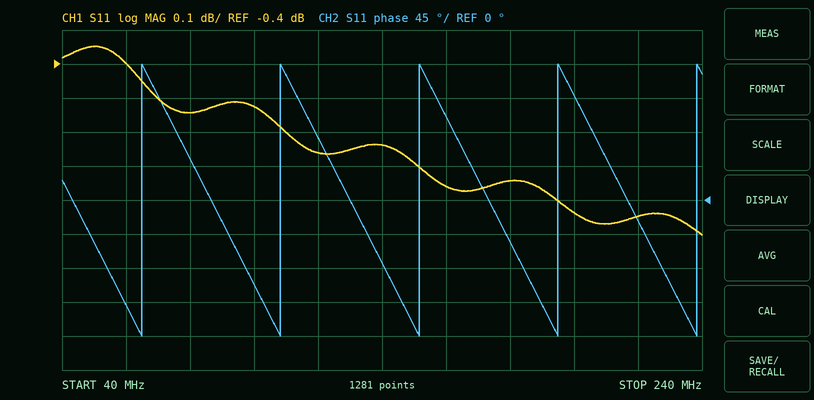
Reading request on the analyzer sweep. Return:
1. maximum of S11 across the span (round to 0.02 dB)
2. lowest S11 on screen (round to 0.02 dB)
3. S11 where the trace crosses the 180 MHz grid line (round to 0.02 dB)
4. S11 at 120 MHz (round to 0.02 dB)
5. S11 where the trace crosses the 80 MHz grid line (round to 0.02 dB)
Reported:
-0.34 dB
-0.90 dB
-0.74 dB
-0.66 dB
-0.54 dB
